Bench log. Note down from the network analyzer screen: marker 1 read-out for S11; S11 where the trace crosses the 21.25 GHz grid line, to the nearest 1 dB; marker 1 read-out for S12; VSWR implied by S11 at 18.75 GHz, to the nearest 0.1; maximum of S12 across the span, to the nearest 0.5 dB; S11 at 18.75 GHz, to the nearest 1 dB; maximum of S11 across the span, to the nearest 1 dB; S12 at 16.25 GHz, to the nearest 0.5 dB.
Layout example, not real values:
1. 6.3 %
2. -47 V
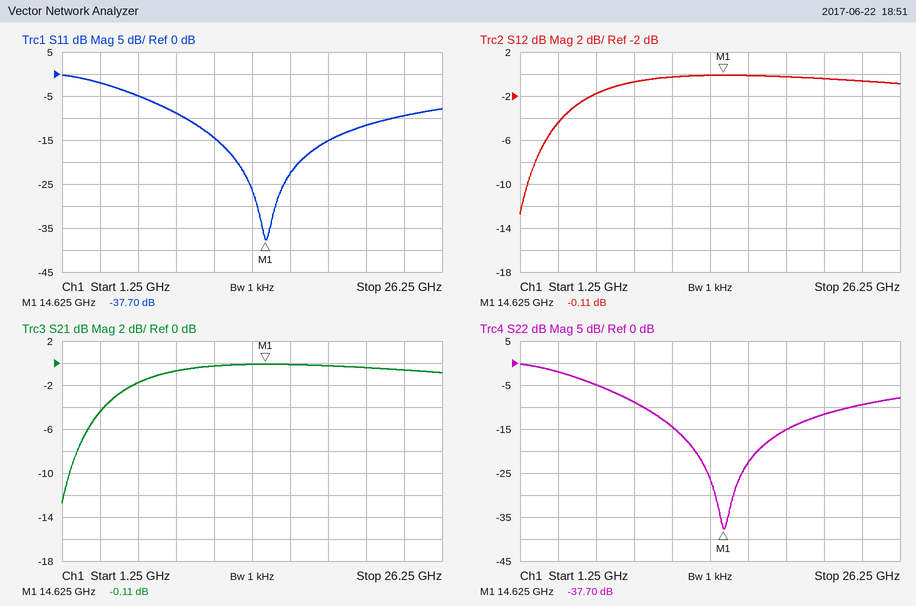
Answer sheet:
1. -37.70 dB
2. -12 dB
3. -0.11 dB
4. 1.4
5. 0.0 dB
6. -15 dB
7. 0 dB
8. 0.0 dB
